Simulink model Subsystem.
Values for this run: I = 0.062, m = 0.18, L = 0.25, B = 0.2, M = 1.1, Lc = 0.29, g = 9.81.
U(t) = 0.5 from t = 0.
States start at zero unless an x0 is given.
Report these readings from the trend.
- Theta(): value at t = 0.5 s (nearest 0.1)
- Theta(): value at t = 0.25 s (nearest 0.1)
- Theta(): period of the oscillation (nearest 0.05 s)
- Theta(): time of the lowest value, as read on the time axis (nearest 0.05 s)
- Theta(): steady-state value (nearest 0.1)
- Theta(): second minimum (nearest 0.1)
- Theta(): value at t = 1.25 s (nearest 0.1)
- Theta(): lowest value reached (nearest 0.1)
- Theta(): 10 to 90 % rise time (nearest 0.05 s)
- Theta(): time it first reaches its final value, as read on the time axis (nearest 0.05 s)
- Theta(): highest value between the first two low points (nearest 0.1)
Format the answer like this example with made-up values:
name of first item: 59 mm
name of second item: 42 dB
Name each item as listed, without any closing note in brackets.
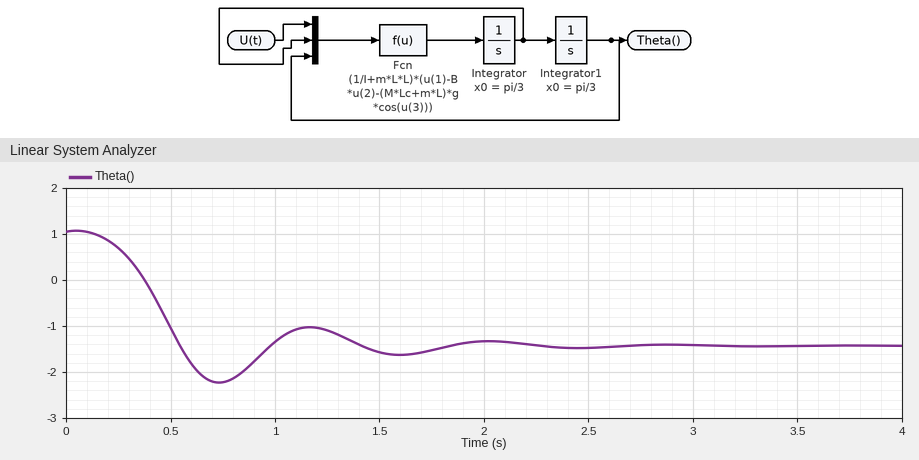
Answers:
Theta(): value at t = 0.5 s: -1.0
Theta(): value at t = 0.25 s: 0.7
Theta(): period of the oscillation: 0.85 s
Theta(): time of the lowest value, as read on the time axis: 0.75 s
Theta(): steady-state value: -1.4
Theta(): second minimum: -1.6
Theta(): value at t = 1.25 s: -1.1
Theta(): lowest value reached: -2.2
Theta(): 10 to 90 % rise time: 0.30 s
Theta(): time it first reaches its final value, as read on the time axis: 0.55 s
Theta(): highest value between the first two low points: -1.0
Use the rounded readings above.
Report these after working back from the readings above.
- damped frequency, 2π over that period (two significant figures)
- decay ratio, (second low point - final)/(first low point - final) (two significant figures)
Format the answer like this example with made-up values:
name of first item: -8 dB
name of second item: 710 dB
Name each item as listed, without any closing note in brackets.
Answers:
damped frequency, 2π over that period: 7.4 rad/s
decay ratio, (second low point - final)/(first low point - final): 0.25
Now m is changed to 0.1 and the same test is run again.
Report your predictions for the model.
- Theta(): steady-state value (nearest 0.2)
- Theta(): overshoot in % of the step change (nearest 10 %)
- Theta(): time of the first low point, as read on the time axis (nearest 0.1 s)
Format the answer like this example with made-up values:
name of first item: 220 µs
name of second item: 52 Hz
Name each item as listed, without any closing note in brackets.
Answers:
Theta(): steady-state value: -1.4
Theta(): overshoot in % of the step change: 30 %
Theta(): time of the first low point, as read on the time axis: 0.8 s
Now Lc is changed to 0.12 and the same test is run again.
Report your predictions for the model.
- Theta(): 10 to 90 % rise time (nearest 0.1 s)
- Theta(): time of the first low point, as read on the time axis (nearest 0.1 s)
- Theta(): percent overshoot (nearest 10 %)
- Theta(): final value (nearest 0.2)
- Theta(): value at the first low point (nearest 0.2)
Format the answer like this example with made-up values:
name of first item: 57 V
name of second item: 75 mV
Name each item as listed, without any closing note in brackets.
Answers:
Theta(): 10 to 90 % rise time: 0.5 s
Theta(): time of the first low point, as read on the time axis: 1.4 s
Theta(): percent overshoot: 20 %
Theta(): final value: -1.2
Theta(): value at the first low point: -1.8
